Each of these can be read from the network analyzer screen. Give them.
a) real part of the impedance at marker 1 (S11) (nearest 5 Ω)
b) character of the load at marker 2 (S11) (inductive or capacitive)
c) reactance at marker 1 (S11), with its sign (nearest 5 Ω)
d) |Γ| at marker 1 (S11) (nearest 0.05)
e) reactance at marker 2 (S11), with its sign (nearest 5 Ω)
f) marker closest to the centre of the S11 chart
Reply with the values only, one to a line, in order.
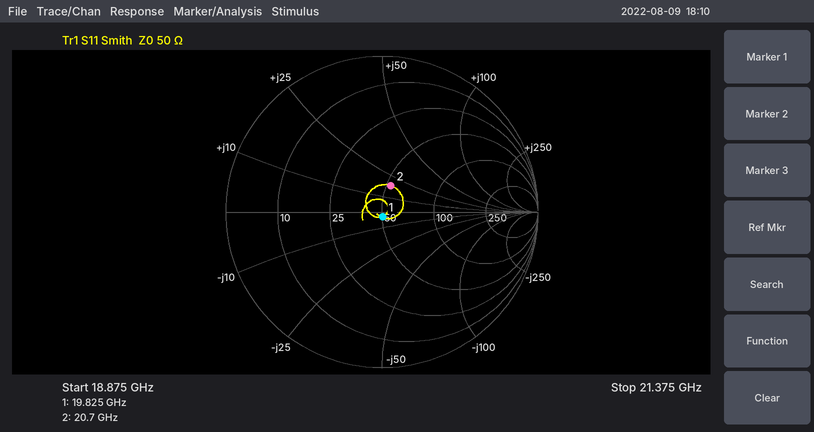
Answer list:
50 Ω
inductive
-5 Ω
0.05
+20 Ω
marker 1
